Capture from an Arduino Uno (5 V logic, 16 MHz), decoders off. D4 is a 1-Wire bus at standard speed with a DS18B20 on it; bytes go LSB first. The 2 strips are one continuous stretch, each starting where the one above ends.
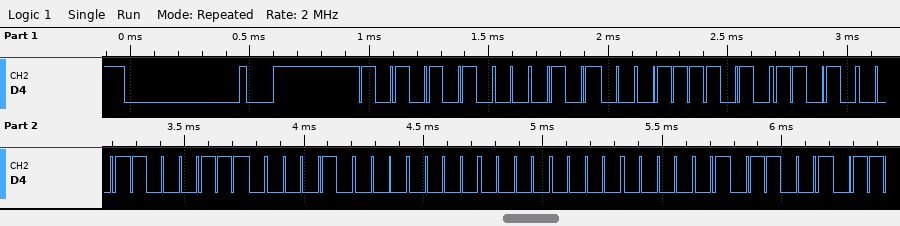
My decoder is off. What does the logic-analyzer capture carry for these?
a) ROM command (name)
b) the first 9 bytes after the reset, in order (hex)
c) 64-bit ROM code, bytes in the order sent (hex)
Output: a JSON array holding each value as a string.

["Match ROM", "55 28 5E 8B 71 08 00 00 9A", "28 5E 8B 71 08 00 00 9A"]
